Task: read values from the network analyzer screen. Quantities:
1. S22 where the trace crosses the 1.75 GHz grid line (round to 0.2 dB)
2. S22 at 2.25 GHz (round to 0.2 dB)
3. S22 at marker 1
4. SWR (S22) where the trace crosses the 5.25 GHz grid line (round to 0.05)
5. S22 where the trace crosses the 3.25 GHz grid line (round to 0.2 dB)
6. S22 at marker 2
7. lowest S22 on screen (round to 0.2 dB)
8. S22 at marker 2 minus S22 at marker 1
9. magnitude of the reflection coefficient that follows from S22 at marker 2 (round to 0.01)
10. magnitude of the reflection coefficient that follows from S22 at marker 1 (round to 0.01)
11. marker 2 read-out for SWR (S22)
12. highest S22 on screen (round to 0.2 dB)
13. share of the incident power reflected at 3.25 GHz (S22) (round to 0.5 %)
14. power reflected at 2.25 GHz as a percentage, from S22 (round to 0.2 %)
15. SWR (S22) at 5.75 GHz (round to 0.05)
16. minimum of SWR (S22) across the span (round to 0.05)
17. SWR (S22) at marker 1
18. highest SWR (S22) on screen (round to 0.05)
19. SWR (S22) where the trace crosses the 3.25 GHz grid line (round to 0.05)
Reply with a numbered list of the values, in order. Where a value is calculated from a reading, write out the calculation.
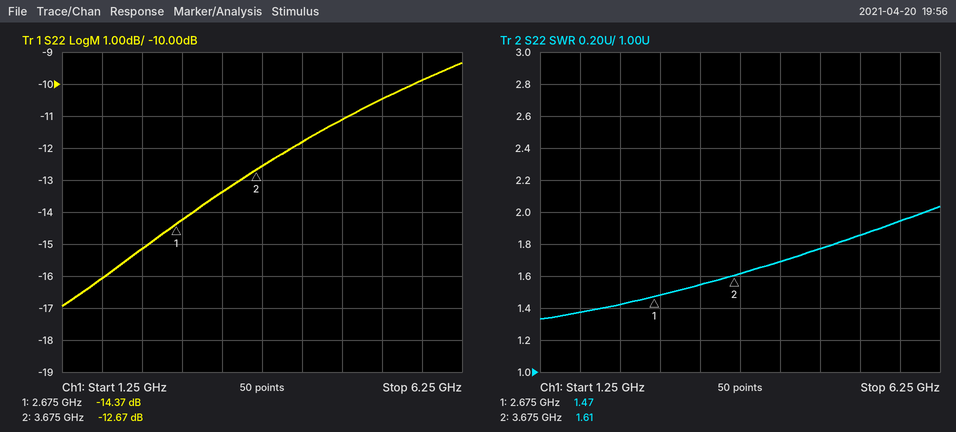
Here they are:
1. -16.0 dB
2. -15.2 dB
3. -14.37 dB
4. 1.85
5. -13.4 dB
6. -12.67 dB
7. -17.0 dB
8. -12.67 − (-14.37) = 1.70 dB
9. 10^(-12.67/20) ≈ 0.23
10. 10^(-14.37/20) ≈ 0.19
11. 1.61
12. -9.4 dB
13. 10^(-13.4/10) ≈ 4.57 %, so 4.5 % to the nearest 0.5 %
14. 10^(-15.2/10) ≈ 3.0 %
15. 1.95
16. 1.35
17. 1.47
18. 2.05
19. 1.55
